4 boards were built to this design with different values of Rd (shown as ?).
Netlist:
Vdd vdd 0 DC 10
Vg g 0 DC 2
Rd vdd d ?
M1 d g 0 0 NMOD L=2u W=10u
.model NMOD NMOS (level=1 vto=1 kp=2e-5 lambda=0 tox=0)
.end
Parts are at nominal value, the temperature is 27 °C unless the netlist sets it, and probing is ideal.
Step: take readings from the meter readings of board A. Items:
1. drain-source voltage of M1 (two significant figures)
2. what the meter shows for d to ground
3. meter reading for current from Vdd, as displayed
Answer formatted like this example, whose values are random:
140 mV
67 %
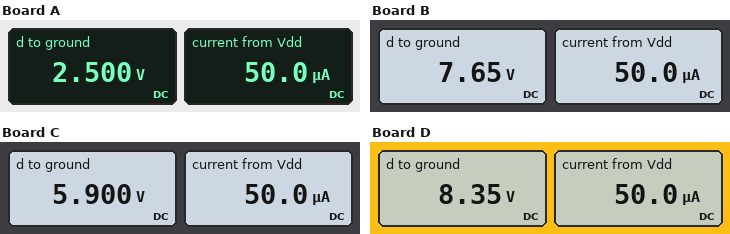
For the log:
2.5 V
2.500 V
50.0 µA
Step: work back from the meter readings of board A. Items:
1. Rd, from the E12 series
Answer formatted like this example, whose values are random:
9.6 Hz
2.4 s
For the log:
150 kΩ
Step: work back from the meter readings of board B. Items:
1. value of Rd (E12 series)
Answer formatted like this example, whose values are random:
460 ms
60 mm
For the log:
47 kΩ
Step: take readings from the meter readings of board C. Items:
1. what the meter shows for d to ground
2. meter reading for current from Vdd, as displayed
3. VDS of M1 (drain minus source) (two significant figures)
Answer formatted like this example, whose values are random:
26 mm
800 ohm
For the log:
5.900 V
50.0 µA
5.9 V
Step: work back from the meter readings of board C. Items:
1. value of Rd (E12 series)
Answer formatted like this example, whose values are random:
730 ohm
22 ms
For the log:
82 kΩ
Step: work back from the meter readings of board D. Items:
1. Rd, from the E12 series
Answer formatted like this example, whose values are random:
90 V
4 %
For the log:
33 kΩ
